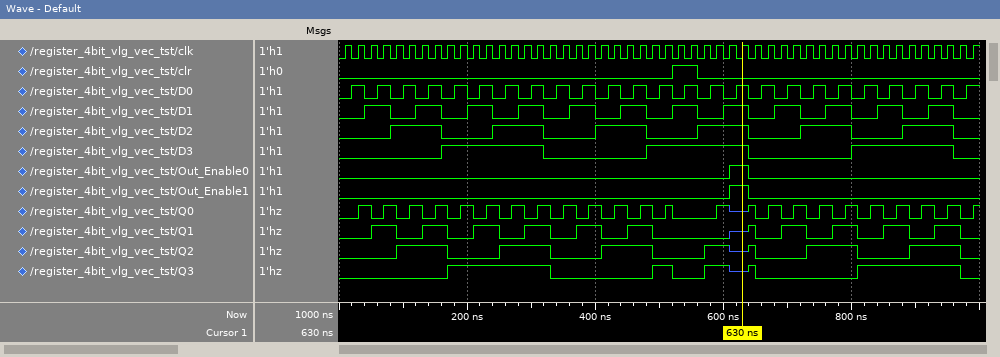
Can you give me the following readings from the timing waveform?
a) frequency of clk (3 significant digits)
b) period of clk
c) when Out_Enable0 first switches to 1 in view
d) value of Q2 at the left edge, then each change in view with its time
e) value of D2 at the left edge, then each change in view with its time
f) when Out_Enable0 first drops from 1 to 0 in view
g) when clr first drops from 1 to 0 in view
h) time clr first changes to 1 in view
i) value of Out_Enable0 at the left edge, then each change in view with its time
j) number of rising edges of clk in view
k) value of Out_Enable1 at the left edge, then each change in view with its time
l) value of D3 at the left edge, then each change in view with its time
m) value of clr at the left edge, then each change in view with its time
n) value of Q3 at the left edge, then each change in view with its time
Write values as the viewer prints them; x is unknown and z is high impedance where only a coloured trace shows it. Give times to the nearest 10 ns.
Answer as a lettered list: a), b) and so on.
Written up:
a) 50.0 MHz
b) 20 ns
c) 610 ns
d) 0, 1 at 90 ns, 0 at 170 ns, 1 at 250 ns, 0 at 330 ns, 1 at 410 ns, 0 at 490 ns, 1 at 570 ns, z at 610 ns, 1 at 640 ns, 0 at 650 ns, 1 at 730 ns, 0 at 810 ns, 1 at 890 ns, 0 at 970 ns
e) 0, 1 at 80 ns, 0 at 160 ns, 1 at 240 ns, 0 at 320 ns, 1 at 400 ns, 0 at 480 ns, 1 at 560 ns, 0 at 640 ns, 1 at 720 ns, 0 at 800 ns, 1 at 880 ns, 0 at 960 ns
f) 640 ns
g) 560 ns
h) 520 ns
i) 0, 1 at 610 ns, 0 at 640 ns
j) 50
k) 0, 1 at 610 ns, 0 at 640 ns
l) 0, 1 at 160 ns, 0 at 320 ns, 1 at 480 ns, 0 at 640 ns, 1 at 800 ns, 0 at 960 ns
m) 0, 1 at 520 ns, 0 at 560 ns
n) 0, 1 at 170 ns, 0 at 330 ns, 1 at 490 ns, 0 at 520 ns, 1 at 570 ns, z at 610 ns, 1 at 640 ns, 0 at 650 ns, 1 at 810 ns, 0 at 970 ns
